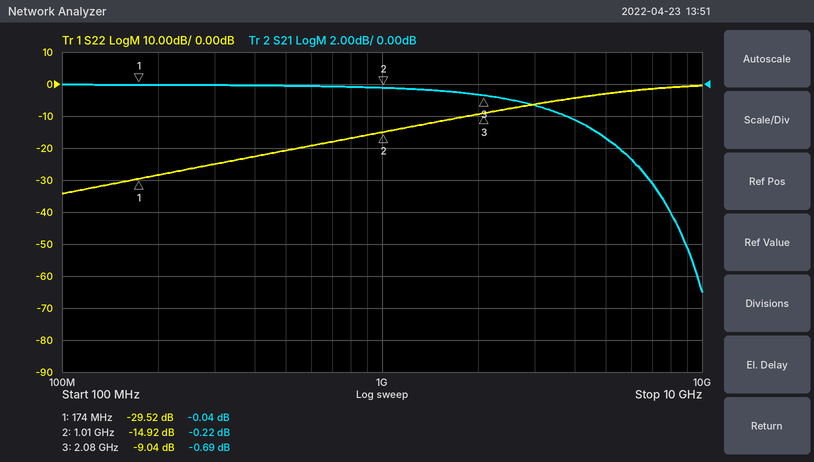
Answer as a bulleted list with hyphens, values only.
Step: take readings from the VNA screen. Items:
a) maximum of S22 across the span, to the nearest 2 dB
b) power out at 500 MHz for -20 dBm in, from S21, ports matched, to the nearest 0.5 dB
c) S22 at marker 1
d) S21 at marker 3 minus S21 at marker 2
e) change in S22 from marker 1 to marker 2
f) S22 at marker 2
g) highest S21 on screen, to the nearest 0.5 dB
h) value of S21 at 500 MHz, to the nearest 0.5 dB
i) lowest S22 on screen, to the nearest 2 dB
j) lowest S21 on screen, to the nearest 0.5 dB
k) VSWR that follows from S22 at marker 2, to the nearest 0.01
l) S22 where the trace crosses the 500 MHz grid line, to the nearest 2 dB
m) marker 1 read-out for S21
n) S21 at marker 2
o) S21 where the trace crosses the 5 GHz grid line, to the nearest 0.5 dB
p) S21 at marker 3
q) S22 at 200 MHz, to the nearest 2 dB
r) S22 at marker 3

- 0 dB
- -20.0 dBm
- -29.52 dB
- -0.47 dB
- 14.60 dB
- -14.92 dB
- 0.0 dB
- 0.0 dB
- -34 dB
- -13.0 dB
- 1.44
- -20 dB
- -0.04 dB
- -0.22 dB
- -3.5 dB
- -0.69 dB
- -28 dB
- -9.04 dB
